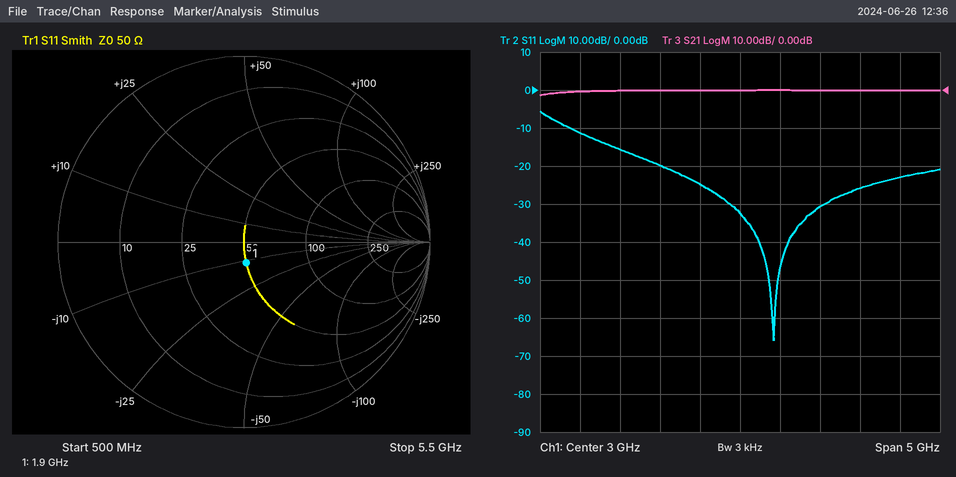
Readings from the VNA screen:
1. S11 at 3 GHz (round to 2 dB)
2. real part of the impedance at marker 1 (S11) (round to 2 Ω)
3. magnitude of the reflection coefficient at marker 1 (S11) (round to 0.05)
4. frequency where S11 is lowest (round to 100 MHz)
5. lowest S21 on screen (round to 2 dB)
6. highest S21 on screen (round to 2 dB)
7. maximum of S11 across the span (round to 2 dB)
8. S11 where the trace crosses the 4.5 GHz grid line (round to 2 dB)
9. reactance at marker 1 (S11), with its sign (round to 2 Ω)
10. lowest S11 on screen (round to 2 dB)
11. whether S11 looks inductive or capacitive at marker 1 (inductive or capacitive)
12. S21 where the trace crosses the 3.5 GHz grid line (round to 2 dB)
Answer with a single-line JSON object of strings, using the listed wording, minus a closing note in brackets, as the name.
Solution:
{"S11 at 3 GHz": "-32 dB", "real part of the impedance at marker 1 (S11)": "50 Ω", "magnitude of the reflection coefficient at marker 1 (S11)": "0.10", "frequency where S11 is lowest": "3.4 GHz", "lowest S21 on screen": "-2 dB", "highest S21 on screen": "0 dB", "maximum of S11 across the span": "-6 dB", "S11 where the trace crosses the 4.5 GHz grid line": "-26 dB", "reactance at marker 1 (S11), with its sign": "-12 Ω", "lowest S11 on screen": "-66 dB", "whether S11 looks inductive or capacitive at marker 1": "capacitive", "S21 where the trace crosses the 3.5 GHz grid line": "0 dB"}
